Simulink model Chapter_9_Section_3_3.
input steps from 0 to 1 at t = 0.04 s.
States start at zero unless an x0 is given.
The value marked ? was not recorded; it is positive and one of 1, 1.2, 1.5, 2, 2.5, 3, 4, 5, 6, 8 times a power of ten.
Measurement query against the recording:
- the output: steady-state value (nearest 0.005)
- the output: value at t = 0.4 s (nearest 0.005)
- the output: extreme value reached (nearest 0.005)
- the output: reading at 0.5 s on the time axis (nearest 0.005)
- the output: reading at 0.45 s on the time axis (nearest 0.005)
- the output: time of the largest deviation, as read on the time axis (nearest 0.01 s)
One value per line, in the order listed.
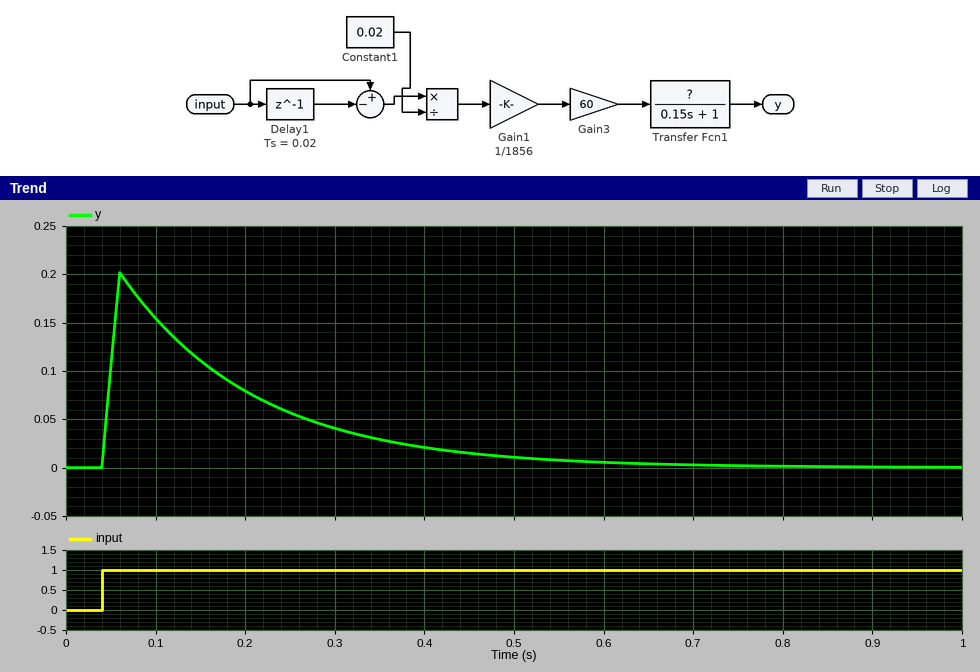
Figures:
0.000
0.020
0.200
0.010
0.015
0.06 s
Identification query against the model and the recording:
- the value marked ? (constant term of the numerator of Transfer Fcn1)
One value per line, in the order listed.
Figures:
1
